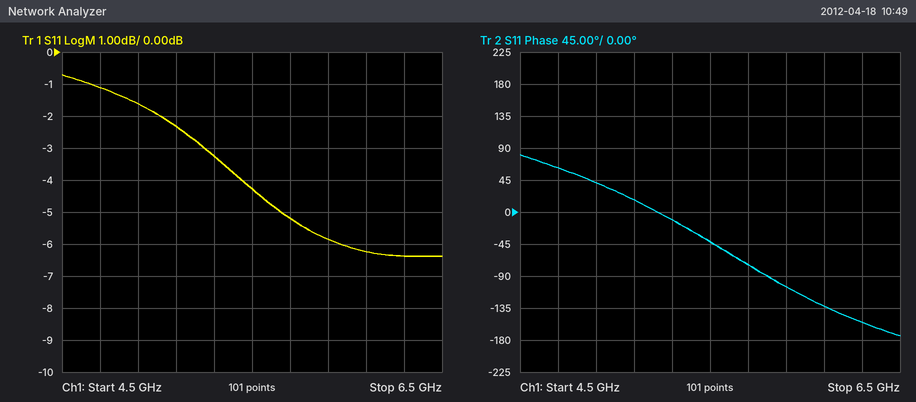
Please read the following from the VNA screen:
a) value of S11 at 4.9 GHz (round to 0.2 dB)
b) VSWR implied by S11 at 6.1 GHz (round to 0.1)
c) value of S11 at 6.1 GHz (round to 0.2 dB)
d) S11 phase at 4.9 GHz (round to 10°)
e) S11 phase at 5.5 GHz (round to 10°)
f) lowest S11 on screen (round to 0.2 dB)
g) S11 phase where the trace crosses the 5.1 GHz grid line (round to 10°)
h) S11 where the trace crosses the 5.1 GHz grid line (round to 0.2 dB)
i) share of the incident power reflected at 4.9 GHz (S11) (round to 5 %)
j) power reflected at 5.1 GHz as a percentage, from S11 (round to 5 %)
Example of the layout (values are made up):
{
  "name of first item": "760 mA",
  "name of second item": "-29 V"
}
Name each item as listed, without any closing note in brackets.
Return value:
{
  "value of S11 at 4.9 GHz": "-1.6 dB",
  "VSWR implied by S11 at 6.1 GHz": "2.9",
  "value of S11 at 6.1 GHz": "-6.2 dB",
  "S11 phase at 4.9 GHz": "40°",
  "S11 phase at 5.5 GHz": "-40°",
  "lowest S11 on screen": "-6.4 dB",
  "S11 phase where the trace crosses the 5.1 GHz grid line": "20°",
  "S11 where the trace crosses the 5.1 GHz grid line": "-2.4 dB",
  "share of the incident power reflected at 4.9 GHz (S11)": "70 %",
  "power reflected at 5.1 GHz as a percentage, from S11": "60 %"
}
